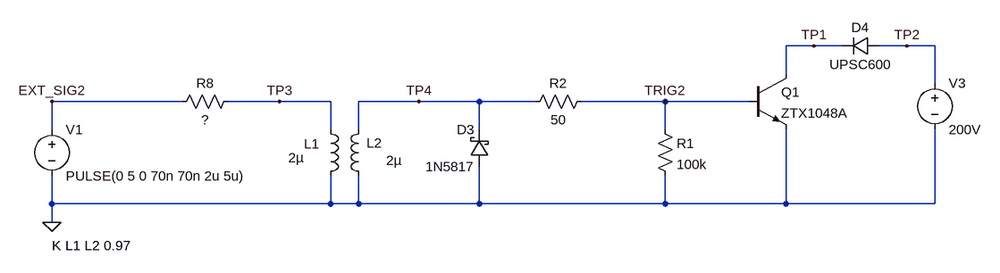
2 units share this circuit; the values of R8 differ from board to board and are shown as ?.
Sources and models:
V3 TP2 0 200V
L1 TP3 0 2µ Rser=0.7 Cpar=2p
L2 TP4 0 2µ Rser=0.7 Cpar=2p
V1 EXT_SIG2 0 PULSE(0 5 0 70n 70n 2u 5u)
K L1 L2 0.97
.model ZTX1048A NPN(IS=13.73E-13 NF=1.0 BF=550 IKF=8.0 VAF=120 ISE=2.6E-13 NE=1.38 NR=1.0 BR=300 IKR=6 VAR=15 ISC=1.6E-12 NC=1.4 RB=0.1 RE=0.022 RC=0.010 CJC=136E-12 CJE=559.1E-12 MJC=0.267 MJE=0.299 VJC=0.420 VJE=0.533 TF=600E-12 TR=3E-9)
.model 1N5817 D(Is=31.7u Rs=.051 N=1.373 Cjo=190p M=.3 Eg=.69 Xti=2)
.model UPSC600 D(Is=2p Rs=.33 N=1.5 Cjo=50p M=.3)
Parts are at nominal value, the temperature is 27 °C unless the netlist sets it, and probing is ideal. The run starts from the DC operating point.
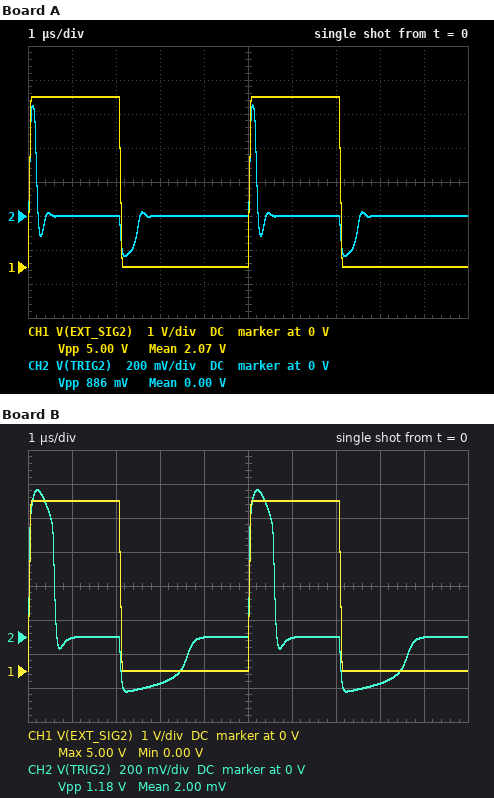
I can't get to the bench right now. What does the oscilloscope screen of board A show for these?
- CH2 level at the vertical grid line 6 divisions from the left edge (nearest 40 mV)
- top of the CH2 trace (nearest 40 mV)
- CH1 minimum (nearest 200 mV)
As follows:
0 V
640 mV
0 V
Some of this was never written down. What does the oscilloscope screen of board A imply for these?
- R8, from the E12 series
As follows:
120 Ω
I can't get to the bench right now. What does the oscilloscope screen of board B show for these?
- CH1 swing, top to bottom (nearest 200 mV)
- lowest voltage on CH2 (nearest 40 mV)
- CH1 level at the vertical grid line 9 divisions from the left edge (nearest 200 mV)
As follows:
5.0 V
-320 mV
0 V
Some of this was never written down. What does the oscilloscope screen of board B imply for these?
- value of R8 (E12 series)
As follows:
18 Ω
